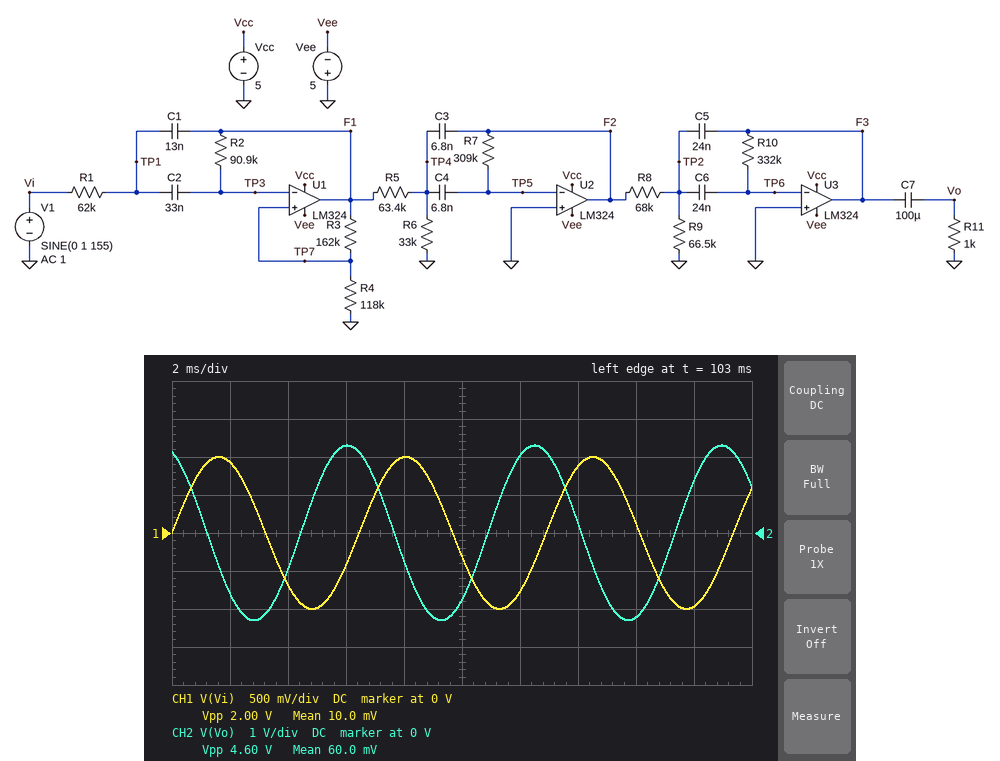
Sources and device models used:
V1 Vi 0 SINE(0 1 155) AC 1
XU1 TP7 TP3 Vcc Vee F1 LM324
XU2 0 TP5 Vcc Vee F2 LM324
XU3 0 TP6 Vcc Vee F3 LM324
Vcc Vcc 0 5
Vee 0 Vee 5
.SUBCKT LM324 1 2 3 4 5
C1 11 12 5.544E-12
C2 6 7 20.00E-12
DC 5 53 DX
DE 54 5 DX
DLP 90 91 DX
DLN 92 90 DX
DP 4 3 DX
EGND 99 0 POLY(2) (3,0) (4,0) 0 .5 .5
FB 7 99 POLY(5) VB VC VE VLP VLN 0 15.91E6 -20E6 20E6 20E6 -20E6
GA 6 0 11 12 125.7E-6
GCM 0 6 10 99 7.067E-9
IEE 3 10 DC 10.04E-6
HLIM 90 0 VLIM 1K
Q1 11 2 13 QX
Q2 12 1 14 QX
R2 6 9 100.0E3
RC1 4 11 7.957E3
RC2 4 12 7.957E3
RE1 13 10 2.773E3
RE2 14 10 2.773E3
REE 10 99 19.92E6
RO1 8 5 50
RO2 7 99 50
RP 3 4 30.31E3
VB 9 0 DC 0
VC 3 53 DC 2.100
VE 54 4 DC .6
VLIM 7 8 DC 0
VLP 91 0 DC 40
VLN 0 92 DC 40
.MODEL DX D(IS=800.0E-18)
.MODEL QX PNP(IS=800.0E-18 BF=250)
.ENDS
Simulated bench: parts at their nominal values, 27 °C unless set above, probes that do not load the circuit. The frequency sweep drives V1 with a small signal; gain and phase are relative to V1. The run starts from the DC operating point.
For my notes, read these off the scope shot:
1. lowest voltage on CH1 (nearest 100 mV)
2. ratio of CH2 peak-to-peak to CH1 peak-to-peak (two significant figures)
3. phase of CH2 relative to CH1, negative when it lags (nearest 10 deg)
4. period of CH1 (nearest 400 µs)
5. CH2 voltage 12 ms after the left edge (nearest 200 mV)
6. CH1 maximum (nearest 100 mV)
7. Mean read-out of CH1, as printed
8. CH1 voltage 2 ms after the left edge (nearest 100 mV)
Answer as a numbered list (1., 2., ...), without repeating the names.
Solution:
1. -1.0 V
2. 2.3
3. 110 deg
4. 6.4 ms
5. 2.0 V
6. 1.0 V
7. 10.0 mV
8. 900 mV
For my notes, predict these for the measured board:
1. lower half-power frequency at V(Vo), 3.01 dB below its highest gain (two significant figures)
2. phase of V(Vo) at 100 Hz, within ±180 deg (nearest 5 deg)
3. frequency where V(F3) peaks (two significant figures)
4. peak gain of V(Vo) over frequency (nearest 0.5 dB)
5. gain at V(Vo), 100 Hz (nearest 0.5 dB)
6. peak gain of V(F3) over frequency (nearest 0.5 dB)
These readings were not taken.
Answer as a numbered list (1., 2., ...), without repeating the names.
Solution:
1. 79 Hz
2. -150 deg
3. 100 Hz
4. 14.5 dB
5. 14.5 dB
6. 14.5 dB
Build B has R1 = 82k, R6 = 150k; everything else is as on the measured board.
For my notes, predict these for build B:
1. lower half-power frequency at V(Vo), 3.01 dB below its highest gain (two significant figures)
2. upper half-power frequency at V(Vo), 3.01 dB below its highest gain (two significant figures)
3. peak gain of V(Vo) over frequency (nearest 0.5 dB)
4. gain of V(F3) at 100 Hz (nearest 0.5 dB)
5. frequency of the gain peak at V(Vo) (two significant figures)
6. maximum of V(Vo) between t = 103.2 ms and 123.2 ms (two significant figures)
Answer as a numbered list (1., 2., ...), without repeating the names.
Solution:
1. 61 Hz
2. 130 Hz
3. 14.0 dB
4. 13.5 dB
5. 82 Hz
6. 2.8 V
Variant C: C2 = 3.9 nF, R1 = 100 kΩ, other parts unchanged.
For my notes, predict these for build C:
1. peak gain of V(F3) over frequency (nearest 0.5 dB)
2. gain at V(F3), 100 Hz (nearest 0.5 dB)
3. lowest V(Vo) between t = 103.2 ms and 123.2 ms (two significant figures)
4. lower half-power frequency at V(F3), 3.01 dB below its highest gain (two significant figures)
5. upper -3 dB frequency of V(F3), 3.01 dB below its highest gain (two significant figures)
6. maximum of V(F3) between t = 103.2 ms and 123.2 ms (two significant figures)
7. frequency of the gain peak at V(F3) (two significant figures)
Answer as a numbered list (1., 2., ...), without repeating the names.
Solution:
1. -8.5 dB
2. -13.5 dB
3. -260 mV
4. 160 Hz
5. 330 Hz
6. 260 mV
7. 260 Hz
